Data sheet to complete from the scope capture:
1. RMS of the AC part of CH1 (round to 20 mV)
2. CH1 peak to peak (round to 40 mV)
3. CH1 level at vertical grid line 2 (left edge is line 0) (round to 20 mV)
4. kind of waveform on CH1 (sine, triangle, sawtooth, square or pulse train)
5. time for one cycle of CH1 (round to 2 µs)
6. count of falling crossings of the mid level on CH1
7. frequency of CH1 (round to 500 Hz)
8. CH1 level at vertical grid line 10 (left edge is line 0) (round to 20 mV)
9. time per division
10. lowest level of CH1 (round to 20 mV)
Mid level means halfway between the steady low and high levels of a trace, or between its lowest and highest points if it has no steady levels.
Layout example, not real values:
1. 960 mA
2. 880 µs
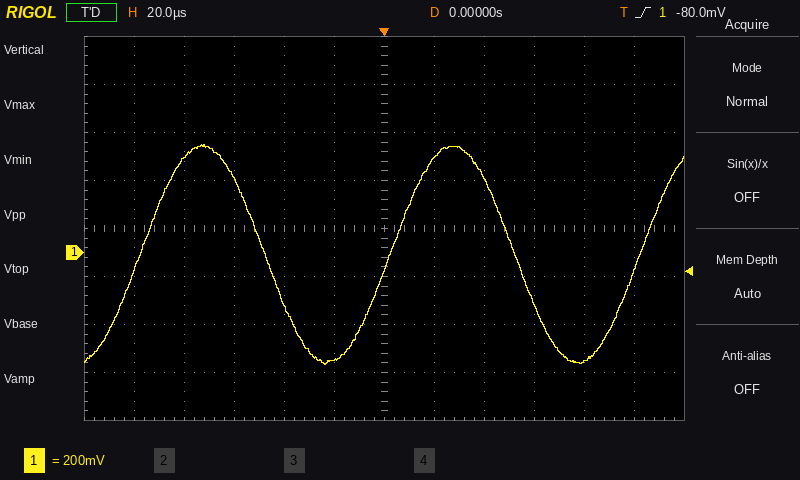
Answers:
1. 320 mV
2. 920 mV
3. 400 mV
4. sine
5. 100 µs
6. 2
7. 10.0 kHz
8. -460 mV
9. 20 µs
10. -460 mV
